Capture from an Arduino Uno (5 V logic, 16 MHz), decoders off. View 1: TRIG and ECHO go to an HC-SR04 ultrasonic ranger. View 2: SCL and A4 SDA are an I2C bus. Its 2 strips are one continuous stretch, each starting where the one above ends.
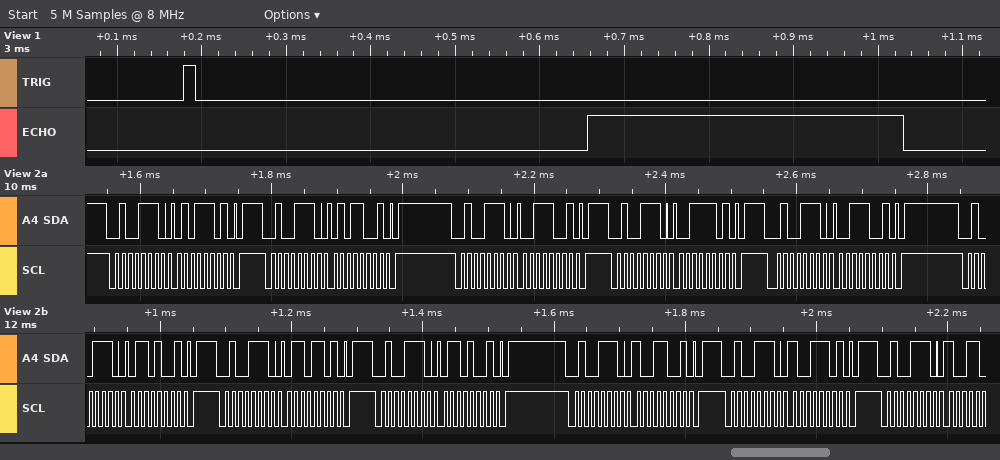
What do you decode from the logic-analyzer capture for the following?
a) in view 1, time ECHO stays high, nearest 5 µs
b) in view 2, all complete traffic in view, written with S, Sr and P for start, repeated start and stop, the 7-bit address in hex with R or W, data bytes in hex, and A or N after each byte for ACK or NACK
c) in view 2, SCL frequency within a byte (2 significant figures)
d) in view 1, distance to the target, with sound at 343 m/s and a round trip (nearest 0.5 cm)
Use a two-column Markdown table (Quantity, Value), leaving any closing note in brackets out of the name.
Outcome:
| Quantity | Value |
|---|---|
| in view 1, time ECHO stays high, nearest 5 µs | 375 µs |
| in view 2, all complete traffic in view, written with S, Sr and P for start, repeated start and stop, the 7-bit address in hex with R or W, data bytes in hex, and A or N after each byte for ACK or NACK | S 27W A 5D A P S 27W A 59 A P S 27W A 39 A P S 27W A 3D A P S 27W A 39 A P S 27W A 69 A P S 27W A 6D A P S 27W A 69 A P S 27W A 99 A P S 27W A 9D A P S 27W A |
| in view 2, SCL frequency within a byte | 100 kHz |
| in view 1, distance to the target, with sound at 343 m/s and a round trip | 6.5 cm |
